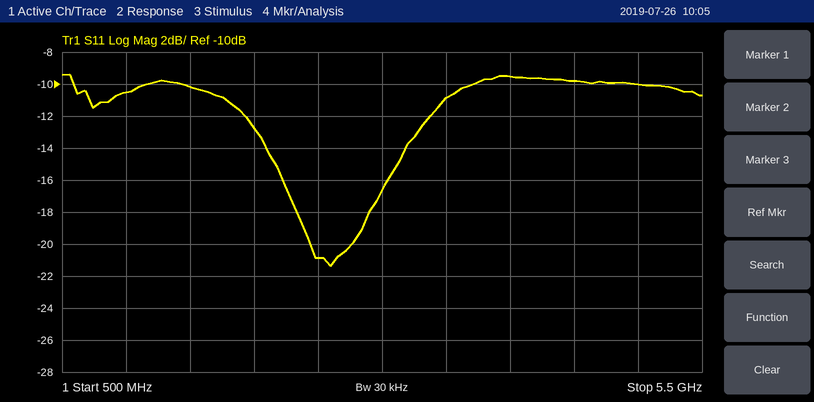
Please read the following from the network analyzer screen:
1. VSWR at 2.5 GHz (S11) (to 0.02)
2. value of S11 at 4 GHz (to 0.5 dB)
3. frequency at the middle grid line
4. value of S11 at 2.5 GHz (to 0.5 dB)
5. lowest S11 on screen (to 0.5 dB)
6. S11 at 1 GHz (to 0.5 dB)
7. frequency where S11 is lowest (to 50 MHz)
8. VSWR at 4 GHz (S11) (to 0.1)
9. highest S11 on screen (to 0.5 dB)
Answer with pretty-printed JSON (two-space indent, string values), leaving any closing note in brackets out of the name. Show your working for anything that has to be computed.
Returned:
{
  "VSWR at 2.5 GHz (S11)": "|Γ| = 10^(-21/20) = 0.0891; VSWR = (1 + 0.0891)/(1 − 0.0891) ≈ 1.20",
  "value of S11 at 4 GHz": "-9.5 dB",
  "frequency at the middle grid line": "3 GHz",
  "value of S11 at 2.5 GHz": "-21.0 dB",
  "lowest S11 on screen": "-21.5 dB",
  "S11 at 1 GHz": "-10.5 dB",
  "frequency where S11 is lowest": "2.60 GHz",
  "VSWR at 4 GHz (S11)": "|Γ| = 10^(-9.5/20) = 0.3350; VSWR = (1 + 0.3350)/(1 − 0.3350) ≈ 2.0",
  "highest S11 on screen": "-9.5 dB"
}
